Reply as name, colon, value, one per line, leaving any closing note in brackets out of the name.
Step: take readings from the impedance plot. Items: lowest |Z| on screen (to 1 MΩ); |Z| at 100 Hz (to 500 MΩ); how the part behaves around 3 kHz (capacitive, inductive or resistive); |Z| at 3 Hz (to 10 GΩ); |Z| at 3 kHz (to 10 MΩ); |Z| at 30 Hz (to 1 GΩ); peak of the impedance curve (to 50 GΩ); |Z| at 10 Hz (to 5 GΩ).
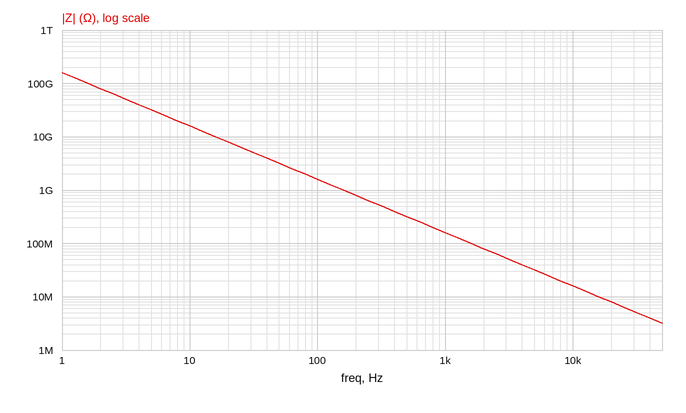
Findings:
lowest |Z| on screen: 3 MΩ
|Z| at 100 Hz: 1.5 GΩ
how the part behaves around 3 kHz: capacitive
|Z| at 3 Hz: 50 GΩ
|Z| at 3 kHz: 50 MΩ
|Z| at 30 Hz: 5 GΩ
peak of the impedance curve: 150 GΩ
|Z| at 10 Hz: 15 GΩ
